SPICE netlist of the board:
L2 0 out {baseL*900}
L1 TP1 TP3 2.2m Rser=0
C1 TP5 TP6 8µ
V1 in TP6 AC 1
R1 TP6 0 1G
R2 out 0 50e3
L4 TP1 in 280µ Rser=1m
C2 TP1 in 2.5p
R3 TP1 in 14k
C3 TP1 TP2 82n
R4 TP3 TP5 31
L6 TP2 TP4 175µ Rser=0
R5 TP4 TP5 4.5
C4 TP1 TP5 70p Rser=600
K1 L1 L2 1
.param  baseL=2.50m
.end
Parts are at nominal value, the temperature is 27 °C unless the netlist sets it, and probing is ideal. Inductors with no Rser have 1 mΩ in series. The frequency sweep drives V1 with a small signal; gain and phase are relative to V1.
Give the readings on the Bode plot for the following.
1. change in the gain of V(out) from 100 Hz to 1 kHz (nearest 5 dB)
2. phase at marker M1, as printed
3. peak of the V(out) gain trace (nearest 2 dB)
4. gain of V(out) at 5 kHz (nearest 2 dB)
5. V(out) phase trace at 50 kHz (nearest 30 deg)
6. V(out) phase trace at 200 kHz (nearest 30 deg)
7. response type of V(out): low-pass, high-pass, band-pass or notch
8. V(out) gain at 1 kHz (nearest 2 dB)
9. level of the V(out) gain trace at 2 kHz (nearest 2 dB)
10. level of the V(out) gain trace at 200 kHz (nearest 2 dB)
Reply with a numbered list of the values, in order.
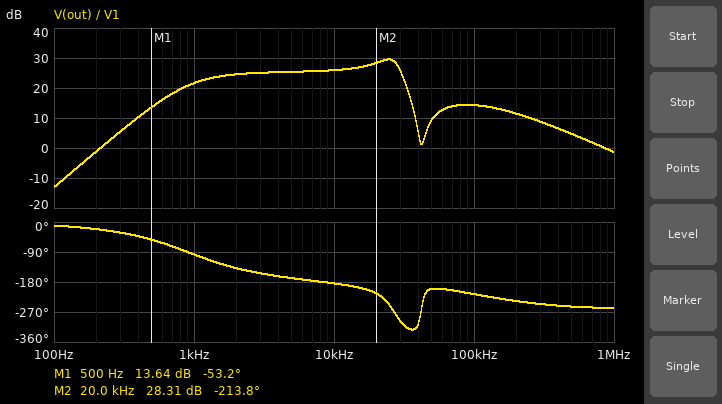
1. 35 dB
2. -53.2 deg
3. 30 dB
4. 26 dB
5. -210 deg
6. -240 deg
7. band-pass
8. 22 dB
9. 24 dB
10. 12 dB
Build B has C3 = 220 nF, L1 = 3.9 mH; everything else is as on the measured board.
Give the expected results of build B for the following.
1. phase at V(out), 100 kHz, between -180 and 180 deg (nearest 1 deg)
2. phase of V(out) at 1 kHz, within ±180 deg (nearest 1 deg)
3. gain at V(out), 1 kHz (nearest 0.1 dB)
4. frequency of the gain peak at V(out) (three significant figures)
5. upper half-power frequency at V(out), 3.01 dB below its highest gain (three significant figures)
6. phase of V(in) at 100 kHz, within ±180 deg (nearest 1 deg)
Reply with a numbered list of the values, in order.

1. 151 deg
2. -113 deg
3. 23.3 dB
4. 15.8 kHz
5. 17.4 kHz
6. 0 deg
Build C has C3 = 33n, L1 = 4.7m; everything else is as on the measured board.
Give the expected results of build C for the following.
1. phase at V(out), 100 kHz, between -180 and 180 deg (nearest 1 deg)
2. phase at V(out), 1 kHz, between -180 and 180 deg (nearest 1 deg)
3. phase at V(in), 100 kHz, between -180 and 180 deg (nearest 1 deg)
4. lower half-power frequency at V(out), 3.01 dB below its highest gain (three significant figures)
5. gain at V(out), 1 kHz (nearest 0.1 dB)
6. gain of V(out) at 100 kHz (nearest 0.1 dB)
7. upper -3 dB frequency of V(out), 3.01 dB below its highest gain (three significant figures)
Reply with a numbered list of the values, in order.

1. 160 deg
2. -119 deg
3. 0 deg
4. 25.6 kHz
5. 23.8 dB
6. 12.2 dB
7. 45.8 kHz
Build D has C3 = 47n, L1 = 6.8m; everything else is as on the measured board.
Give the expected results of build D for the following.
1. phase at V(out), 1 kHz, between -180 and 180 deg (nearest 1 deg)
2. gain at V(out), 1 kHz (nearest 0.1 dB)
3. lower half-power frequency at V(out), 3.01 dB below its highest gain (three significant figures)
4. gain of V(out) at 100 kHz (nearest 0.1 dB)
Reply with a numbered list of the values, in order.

1. -133 deg
2. 23.9 dB
3. 28.0 kHz
4. 12.7 dB
